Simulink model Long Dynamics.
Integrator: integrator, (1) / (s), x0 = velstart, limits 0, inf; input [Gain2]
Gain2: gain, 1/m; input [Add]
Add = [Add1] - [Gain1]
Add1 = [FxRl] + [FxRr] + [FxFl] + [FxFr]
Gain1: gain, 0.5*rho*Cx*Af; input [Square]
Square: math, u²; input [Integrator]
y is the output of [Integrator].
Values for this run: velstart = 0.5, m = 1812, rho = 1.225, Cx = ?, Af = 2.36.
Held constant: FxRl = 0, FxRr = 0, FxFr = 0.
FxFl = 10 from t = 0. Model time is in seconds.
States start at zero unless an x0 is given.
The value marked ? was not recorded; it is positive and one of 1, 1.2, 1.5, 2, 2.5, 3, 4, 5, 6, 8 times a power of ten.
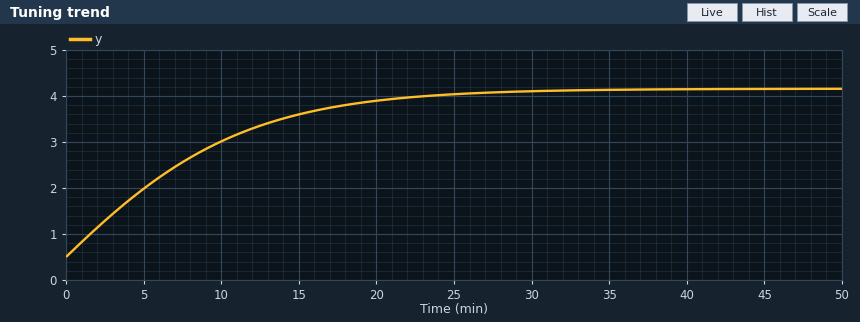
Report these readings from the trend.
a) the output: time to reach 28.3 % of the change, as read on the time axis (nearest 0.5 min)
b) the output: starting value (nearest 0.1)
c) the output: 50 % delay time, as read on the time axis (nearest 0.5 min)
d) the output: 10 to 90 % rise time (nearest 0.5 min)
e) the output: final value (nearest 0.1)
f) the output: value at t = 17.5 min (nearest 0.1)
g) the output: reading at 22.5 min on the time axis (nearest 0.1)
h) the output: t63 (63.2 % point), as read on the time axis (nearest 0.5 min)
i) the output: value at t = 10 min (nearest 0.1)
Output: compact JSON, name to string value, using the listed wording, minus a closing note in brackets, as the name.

{"the output: time to reach 28.3 % of the change, as read on the time axis": "3.5 min", "the output: starting value": "0.5", "the output: 50 % delay time, as read on the time axis": "6.5 min", "the output: 10 to 90 % rise time": "16.5 min", "the output: final value": "4.2", "the output: value at t = 17.5 min": "3.8", "the output: reading at 22.5 min on the time axis": "4.0", "the output: t63 (63.2 % point), as read on the time axis": "9.0 min", "the output: value at t = 10 min": "3.0"}
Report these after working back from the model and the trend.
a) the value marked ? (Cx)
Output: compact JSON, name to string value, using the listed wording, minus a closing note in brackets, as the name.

{"the value marked ?": "0.4"}
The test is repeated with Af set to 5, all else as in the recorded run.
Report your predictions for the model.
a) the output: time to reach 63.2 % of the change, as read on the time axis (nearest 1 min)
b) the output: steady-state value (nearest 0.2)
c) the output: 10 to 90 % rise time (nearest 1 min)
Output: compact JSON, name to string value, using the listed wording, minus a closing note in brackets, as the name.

{"the output: time to reach 63.2 % of the change, as read on the time axis": "6 min", "the output: steady-state value": "2.8", "the output: 10 to 90 % rise time": "11 min"}
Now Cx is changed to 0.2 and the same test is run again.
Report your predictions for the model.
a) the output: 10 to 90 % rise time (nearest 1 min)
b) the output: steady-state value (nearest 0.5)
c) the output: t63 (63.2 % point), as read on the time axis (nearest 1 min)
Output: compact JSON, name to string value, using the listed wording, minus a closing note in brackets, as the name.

{"the output: 10 to 90 % rise time": "24 min", "the output: steady-state value": "6.0", "the output: t63 (63.2 % point), as read on the time axis": "13 min"}
